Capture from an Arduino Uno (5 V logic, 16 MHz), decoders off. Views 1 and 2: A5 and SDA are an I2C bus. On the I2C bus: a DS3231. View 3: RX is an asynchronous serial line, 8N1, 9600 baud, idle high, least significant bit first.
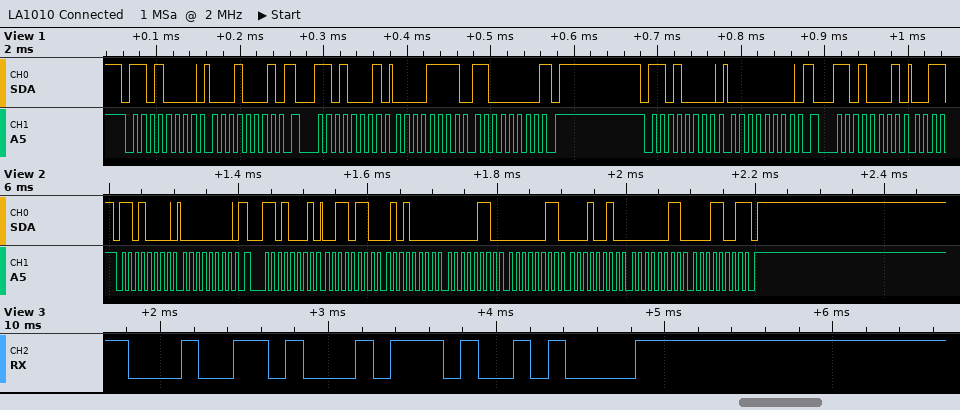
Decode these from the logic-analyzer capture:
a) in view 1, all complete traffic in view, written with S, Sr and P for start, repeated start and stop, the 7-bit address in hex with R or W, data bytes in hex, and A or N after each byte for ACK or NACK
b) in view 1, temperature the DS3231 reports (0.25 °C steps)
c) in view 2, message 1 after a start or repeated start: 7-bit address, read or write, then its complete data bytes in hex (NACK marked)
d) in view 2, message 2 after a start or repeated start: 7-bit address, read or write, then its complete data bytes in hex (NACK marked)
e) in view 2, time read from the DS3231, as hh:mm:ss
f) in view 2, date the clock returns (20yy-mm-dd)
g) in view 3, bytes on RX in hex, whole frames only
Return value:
S 68W A 11 A Sr 68R A 0F A C0 N P S 68W A 00 A Sr 68R A
15.75 °C
0x68 write: 00
0x68 read: 36 50 06 03 12 03 19 NACK
06:50:36
2019-03-12
64 74 0A
